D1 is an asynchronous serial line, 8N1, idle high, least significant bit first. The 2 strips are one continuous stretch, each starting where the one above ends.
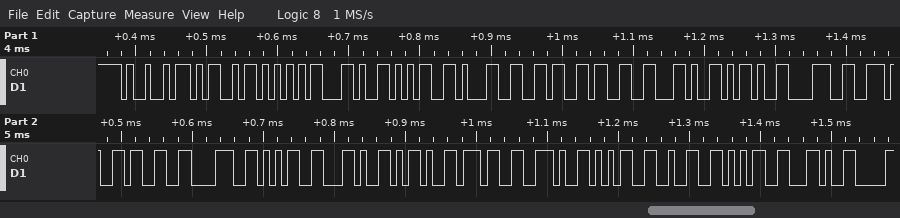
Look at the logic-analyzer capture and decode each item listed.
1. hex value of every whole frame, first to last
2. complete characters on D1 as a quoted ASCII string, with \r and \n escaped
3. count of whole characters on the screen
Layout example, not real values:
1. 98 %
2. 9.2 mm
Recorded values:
1. 0x49 0x4D 0x55 0x2C 0x35 0x31 0x36 0x33 0x2C 0x2D 0x38 0x2E 0x33 0x38 0x35 0x2C 0x2D 0x37 0x2E 0x35 0x32 0x35 0x2C
2. "IMU,5163,-8.385,-7.525,"
3. 23
